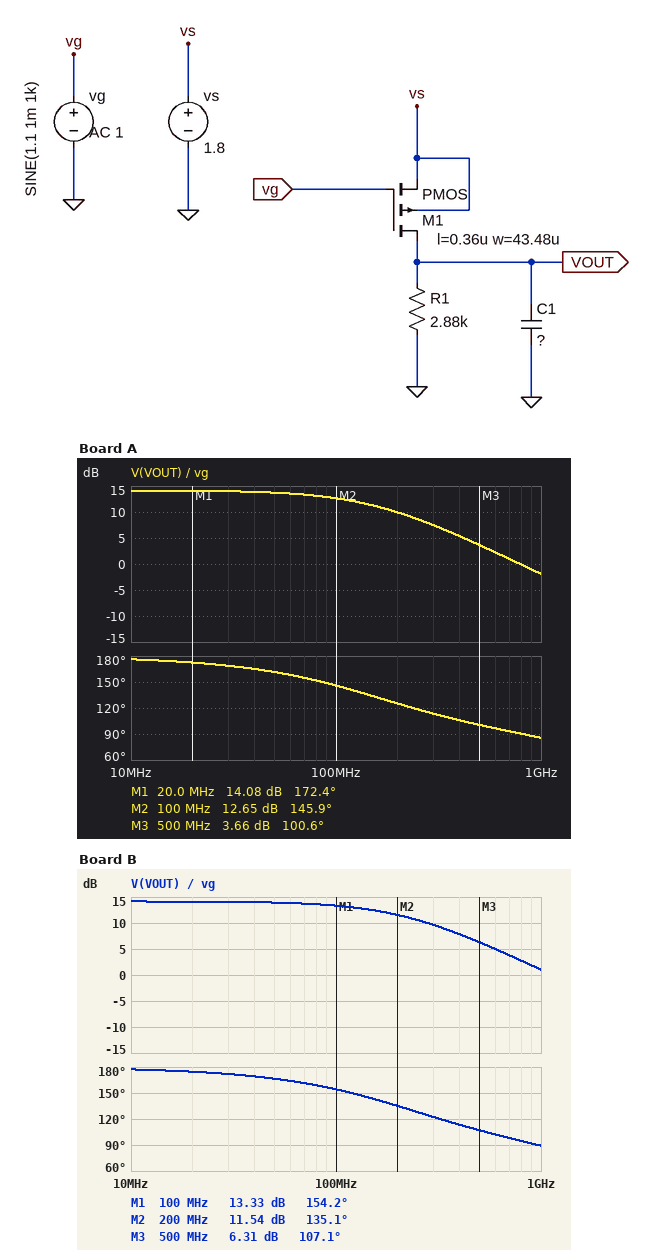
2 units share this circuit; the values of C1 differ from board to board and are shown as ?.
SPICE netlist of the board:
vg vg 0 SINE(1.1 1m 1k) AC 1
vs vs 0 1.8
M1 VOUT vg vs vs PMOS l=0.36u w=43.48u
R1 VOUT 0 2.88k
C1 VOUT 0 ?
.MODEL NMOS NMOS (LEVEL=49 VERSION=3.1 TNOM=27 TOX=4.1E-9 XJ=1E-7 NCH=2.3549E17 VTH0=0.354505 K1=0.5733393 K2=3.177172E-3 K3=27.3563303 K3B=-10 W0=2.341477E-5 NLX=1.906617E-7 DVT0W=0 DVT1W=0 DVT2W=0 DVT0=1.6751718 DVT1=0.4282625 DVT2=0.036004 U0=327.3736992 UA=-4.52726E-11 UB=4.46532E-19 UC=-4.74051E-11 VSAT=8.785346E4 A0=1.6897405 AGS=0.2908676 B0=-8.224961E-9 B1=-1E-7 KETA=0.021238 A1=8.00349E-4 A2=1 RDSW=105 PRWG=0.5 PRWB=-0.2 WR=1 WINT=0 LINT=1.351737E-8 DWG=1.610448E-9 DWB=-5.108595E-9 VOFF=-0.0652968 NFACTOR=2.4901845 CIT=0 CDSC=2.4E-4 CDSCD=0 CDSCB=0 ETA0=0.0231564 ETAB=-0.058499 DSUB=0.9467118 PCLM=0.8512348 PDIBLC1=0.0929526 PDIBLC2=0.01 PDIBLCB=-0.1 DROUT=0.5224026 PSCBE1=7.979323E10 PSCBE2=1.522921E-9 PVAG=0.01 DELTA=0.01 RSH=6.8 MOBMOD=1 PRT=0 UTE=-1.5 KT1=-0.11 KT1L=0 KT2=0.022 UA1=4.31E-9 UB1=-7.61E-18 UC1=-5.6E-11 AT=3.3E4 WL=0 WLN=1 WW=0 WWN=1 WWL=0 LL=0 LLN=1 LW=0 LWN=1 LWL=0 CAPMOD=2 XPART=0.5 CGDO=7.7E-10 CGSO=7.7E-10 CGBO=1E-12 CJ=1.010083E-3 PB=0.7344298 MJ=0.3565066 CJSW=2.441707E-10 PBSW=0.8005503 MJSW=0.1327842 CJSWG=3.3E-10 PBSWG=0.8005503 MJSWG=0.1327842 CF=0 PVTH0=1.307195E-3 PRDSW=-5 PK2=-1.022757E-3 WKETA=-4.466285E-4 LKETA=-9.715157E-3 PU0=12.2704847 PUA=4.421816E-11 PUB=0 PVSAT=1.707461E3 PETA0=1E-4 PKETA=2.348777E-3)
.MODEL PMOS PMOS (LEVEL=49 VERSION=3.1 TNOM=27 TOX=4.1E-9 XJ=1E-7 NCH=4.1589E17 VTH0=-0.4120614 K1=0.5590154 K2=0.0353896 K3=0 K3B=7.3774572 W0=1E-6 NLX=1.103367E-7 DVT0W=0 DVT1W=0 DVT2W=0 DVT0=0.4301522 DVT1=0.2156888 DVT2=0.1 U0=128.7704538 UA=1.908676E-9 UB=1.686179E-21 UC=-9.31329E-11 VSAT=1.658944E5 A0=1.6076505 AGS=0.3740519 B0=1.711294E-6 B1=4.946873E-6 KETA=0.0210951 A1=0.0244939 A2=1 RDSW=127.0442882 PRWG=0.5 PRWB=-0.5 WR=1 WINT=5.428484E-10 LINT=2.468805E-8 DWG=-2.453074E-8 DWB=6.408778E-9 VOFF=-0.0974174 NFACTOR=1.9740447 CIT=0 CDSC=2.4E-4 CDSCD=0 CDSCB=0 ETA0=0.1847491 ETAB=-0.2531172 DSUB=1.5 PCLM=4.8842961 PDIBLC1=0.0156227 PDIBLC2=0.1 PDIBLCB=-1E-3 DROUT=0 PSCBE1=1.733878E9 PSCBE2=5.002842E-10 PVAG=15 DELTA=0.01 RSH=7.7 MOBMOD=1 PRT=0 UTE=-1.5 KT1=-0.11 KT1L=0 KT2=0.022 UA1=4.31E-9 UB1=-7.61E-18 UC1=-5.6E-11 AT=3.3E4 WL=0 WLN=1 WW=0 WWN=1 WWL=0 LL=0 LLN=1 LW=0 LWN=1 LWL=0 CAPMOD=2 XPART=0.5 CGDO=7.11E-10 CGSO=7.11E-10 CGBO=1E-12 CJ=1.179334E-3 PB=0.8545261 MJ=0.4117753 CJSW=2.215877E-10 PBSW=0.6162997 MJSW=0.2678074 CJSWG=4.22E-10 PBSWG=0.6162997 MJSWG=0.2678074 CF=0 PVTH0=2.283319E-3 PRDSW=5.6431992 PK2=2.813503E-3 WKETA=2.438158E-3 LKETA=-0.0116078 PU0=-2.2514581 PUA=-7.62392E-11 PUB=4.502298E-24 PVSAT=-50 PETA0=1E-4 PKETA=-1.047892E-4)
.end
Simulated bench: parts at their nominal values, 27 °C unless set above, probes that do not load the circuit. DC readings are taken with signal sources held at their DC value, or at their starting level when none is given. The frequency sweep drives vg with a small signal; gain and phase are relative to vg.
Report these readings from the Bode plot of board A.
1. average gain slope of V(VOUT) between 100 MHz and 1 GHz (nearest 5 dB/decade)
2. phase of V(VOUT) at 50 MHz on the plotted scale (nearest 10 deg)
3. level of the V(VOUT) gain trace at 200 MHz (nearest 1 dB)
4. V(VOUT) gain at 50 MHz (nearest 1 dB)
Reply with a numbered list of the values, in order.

1. -15 dB/decade
2. 160 deg
3. 10 dB
4. 14 dB
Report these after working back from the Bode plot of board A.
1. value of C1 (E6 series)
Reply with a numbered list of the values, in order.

1. 330 fF
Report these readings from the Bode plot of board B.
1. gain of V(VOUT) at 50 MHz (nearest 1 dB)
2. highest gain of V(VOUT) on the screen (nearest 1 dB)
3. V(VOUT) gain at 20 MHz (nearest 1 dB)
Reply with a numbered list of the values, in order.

1. 14 dB
2. 14 dB
3. 14 dB
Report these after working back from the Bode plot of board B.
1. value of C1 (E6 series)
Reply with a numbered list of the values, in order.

1. 220 fF
